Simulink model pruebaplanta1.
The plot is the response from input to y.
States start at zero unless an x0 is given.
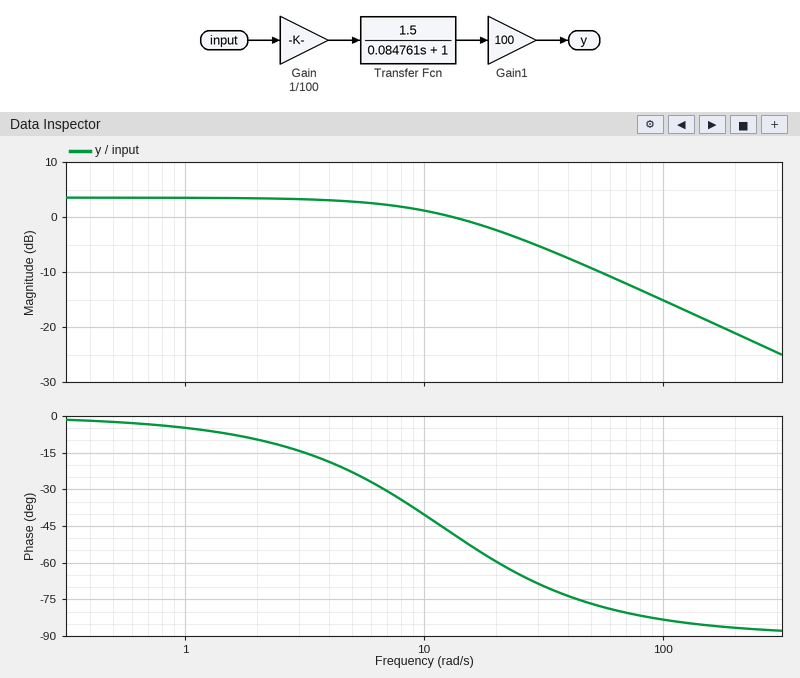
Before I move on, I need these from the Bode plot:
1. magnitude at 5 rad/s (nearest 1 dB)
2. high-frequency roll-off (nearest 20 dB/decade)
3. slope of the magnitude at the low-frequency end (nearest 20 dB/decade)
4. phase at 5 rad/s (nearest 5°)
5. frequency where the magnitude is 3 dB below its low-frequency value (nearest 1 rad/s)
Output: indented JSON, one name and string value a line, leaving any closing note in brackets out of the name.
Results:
{
  "magnitude at 5 rad/s": "3 dB",
  "high-frequency roll-off": "-20 dB/decade",
  "slope of the magnitude at the low-frequency end": "0 dB/decade",
  "phase at 5 rad/s": "-25°",
  "frequency where the magnitude is 3 dB below its low-frequency value": "12 rad/s"
}
